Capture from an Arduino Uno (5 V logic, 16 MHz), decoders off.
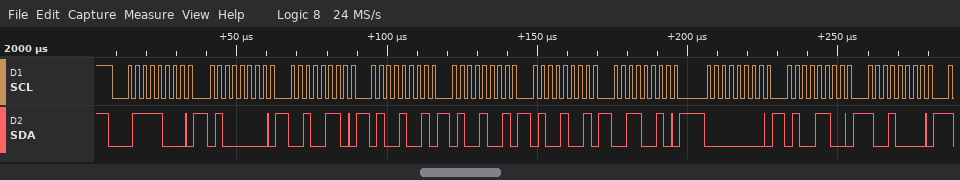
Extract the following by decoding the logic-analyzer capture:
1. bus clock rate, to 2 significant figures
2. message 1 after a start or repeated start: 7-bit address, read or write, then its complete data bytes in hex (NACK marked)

400 kHz
0x3C write: 40 26 49 49 49 32 00 4C 90
